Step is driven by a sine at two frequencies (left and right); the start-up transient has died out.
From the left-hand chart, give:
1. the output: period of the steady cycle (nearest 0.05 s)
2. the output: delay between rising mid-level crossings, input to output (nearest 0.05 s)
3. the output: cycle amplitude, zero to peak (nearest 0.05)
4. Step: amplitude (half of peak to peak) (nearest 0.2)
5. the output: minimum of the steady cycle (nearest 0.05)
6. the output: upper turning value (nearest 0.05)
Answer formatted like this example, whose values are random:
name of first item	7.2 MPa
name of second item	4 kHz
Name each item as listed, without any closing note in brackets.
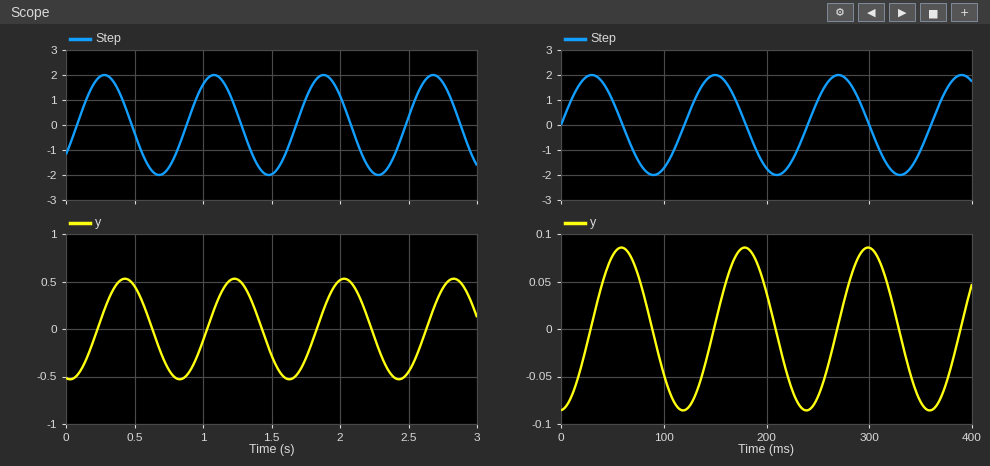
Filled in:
the output: period of the steady cycle	0.80 s
the output: delay between rising mid-level crossings, input to output	0.15 s
the output: cycle amplitude, zero to peak	0.55
Step: amplitude (half of peak to peak)	2.0
the output: minimum of the steady cycle	-0.55
the output: upper turning value	0.55
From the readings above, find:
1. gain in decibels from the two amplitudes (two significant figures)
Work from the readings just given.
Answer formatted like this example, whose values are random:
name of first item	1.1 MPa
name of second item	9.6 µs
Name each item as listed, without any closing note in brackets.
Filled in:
gain in decibels from the two amplitudes	-11 dB
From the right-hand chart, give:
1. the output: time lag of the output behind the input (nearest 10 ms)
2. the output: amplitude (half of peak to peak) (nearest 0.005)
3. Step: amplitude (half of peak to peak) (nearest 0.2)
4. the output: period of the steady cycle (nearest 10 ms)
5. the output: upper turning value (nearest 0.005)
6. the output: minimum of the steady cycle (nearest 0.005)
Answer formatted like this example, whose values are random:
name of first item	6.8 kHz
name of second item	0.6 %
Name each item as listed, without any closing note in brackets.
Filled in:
the output: time lag of the output behind the input	30 ms
the output: amplitude (half of peak to peak)	0.085
Step: amplitude (half of peak to peak)	2.0
the output: period of the steady cycle	120 ms
the output: upper turning value	0.085
the output: minimum of the steady cycle	-0.085
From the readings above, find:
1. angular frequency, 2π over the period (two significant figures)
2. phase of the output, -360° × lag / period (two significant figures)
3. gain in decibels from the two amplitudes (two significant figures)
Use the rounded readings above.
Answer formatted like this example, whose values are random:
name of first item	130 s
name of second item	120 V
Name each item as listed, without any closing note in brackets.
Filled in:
angular frequency, 2π over the period	0.052 rad/ms
phase of the output, -360° × lag / period	-90°
gain in decibels from the two amplitudes	-27 dB
